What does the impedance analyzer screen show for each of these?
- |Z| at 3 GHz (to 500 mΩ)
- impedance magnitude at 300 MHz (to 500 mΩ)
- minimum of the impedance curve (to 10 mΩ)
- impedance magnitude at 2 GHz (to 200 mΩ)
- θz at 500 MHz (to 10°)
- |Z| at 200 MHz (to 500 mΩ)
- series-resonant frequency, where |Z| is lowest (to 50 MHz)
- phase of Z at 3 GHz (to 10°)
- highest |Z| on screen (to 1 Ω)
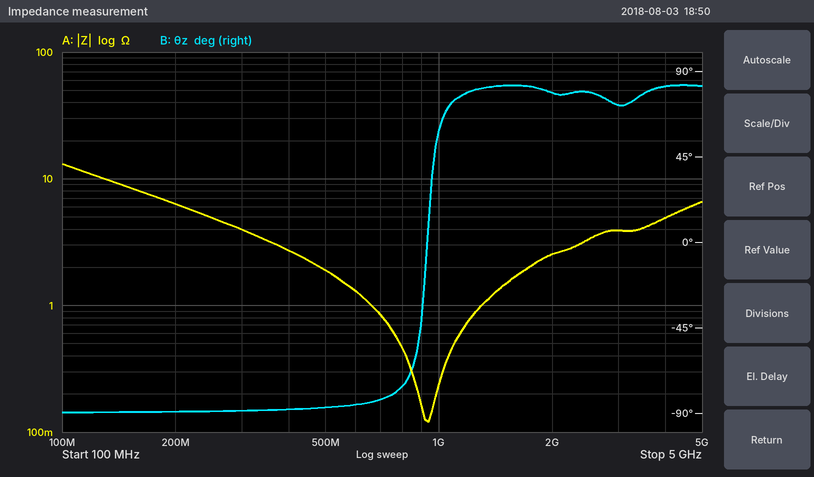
4.0 Ω
4.0 Ω
120 mΩ
2.6 Ω
-90°
6.5 Ω
950 MHz
70°
13 Ω
